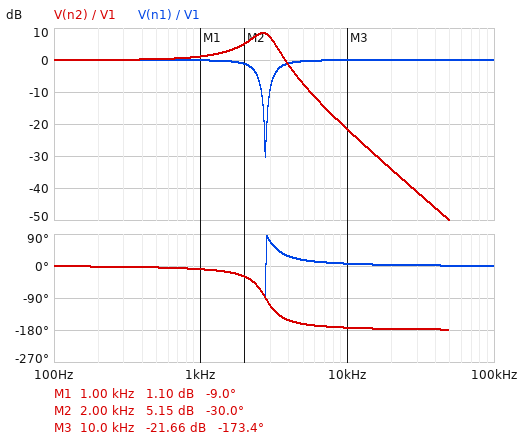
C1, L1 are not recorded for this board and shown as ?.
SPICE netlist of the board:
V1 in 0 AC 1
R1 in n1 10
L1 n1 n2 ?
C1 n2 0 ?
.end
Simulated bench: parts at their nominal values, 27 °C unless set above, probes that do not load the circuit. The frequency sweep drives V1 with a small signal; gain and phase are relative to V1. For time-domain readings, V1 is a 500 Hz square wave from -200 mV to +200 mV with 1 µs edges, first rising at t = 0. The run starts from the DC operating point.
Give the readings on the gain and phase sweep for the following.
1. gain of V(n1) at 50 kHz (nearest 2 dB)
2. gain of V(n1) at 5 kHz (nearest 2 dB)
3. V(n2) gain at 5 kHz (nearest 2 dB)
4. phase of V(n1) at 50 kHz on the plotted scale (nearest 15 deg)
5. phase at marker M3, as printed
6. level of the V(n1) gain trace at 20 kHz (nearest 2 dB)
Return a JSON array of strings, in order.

["0 dB", "0 dB", "-8 dB", "0 deg", "-173.4 deg", "0 dB"]
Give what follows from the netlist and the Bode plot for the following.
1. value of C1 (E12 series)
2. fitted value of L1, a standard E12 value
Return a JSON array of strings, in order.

["2.2 µF", "1.5 mH"]
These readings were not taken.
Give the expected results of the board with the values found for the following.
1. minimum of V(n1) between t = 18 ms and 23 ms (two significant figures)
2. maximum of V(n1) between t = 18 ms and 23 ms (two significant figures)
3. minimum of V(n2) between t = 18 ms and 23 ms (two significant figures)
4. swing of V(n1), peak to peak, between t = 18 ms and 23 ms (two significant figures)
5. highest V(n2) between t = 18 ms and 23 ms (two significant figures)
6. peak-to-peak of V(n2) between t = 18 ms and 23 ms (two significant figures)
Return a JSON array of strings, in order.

["-260 mV", "260 mV", "-420 mV", "530 mV", "420 mV", "840 mV"]
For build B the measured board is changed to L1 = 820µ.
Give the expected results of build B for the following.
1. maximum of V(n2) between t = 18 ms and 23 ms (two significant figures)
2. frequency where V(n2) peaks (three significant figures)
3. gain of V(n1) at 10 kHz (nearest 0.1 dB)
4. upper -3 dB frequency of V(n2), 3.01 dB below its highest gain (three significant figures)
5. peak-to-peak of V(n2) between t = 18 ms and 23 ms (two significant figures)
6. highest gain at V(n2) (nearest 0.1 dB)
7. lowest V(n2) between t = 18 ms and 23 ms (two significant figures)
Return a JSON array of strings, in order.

["370 mV", "3.49 kHz", "-0.2 dB", "4.38 kHz", "750 mV", "6.0 dB", "-370 mV"]
